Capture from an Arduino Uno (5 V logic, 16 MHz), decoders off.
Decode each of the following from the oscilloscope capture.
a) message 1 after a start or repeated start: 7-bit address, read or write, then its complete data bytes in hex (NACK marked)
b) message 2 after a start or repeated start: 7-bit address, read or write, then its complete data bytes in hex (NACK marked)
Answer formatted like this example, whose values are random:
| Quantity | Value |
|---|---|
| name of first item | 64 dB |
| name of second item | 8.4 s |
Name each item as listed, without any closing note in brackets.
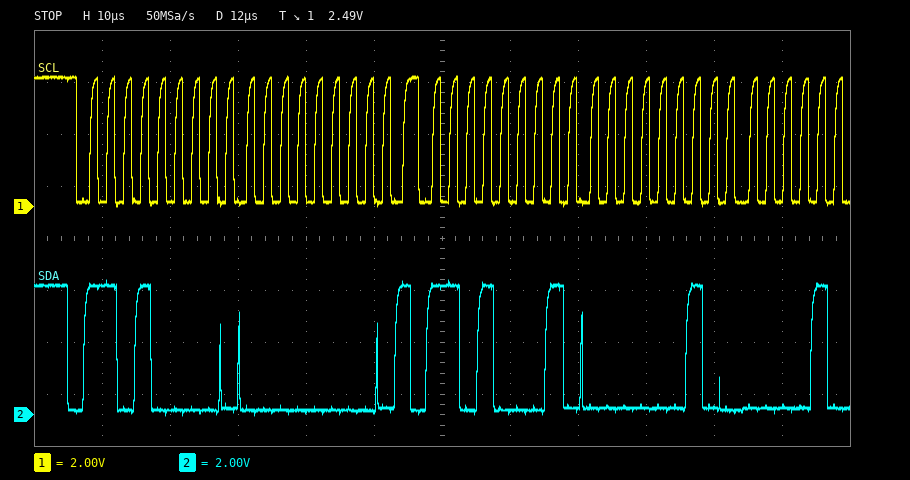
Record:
| Quantity | Value |
|---|---|
| message 1 after a start or repeated start: 7-bit address, read or write, then its complete data bytes in hex | 0x68 write: 00 |
| message 2 after a start or repeated start: 7-bit address, read or write, then its complete data bytes in hex | 0x68 read: 02 |
